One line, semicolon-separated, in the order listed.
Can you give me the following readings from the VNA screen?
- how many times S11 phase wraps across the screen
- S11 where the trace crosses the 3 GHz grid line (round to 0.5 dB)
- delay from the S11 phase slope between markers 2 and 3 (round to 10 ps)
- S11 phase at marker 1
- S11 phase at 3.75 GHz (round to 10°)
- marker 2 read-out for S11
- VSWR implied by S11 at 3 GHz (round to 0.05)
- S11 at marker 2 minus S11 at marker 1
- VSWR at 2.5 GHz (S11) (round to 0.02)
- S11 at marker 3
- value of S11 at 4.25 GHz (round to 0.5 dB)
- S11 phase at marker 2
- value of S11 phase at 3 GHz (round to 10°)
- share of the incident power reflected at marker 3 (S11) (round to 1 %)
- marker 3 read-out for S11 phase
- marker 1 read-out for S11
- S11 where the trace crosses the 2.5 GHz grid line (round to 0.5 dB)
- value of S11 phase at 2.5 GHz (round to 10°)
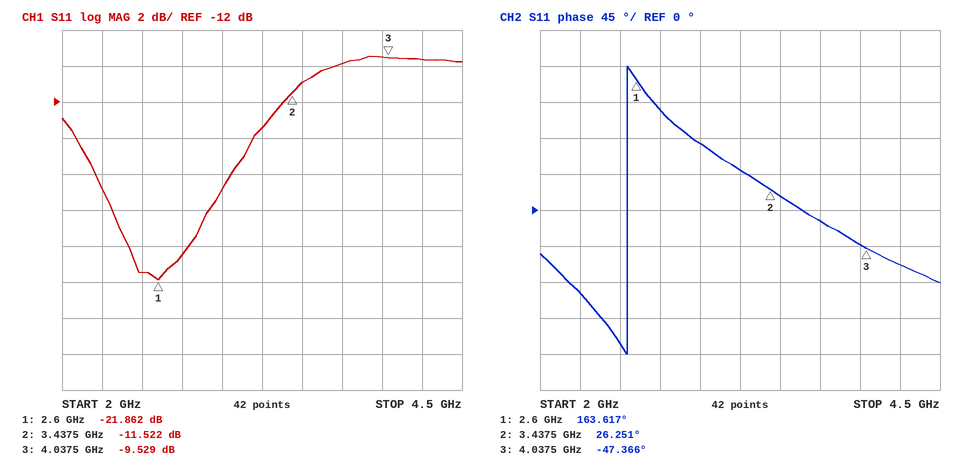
1; -17.0 dB; 340 ps; 163.617°; -10°; -11.522 dB; 1.35; 10.340 dB; 1.18; -9.529 dB; -9.5 dB; 26.251°; 80°; 11 %; -47.366°; -21.862 dB; -21.5 dB; -170°
